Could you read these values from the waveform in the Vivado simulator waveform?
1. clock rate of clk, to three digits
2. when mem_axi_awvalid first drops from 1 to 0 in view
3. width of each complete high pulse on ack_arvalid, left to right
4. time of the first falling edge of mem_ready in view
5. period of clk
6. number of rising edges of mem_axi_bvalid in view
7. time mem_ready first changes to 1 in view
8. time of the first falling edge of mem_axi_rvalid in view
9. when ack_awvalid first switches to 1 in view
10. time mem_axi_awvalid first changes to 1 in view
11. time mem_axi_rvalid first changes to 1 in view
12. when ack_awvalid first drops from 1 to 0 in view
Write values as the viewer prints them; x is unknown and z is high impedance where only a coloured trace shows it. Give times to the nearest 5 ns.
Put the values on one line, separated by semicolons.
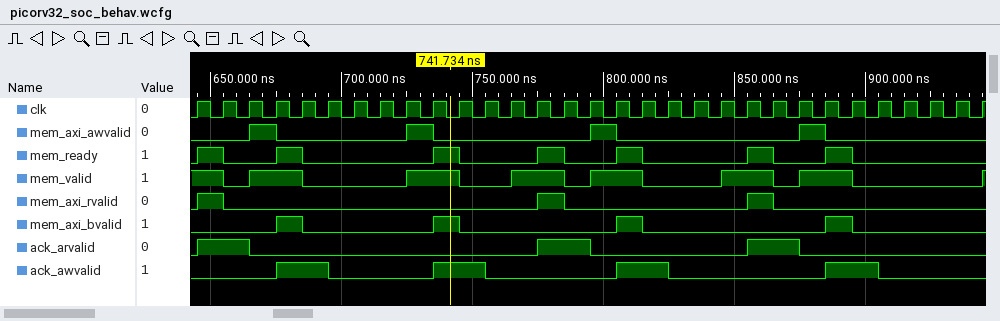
100 MHz; 675 ns; 20 ns, 20 ns, 20 ns; 655 ns; 10 ns; 4; 645 ns; 655 ns; 675 ns; 665 ns; 645 ns; 695 ns
